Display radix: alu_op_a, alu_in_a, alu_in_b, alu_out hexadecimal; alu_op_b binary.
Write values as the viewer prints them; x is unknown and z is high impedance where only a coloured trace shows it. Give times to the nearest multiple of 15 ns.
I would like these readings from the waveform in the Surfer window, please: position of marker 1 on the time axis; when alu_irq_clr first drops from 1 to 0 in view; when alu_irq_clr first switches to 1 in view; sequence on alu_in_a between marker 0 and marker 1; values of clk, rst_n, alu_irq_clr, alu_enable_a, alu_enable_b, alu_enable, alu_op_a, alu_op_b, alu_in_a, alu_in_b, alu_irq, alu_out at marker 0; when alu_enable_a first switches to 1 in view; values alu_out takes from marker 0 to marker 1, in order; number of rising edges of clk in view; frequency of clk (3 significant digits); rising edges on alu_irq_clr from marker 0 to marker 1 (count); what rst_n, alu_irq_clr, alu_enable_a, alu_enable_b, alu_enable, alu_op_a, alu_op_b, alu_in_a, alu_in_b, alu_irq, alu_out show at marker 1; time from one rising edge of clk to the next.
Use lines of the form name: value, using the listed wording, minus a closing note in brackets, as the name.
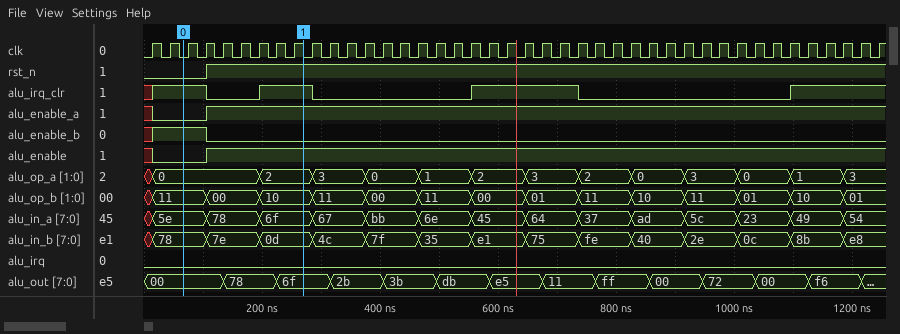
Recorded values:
position of marker 1 on the time axis: 270 ns
when alu_irq_clr first drops from 1 to 0 in view: 105 ns
when alu_irq_clr first switches to 1 in view: 15 ns
sequence on alu_in_a between marker 0 and marker 1: 5e, 78, 6f
values of clk, rst_n, alu_irq_clr, alu_enable_a, alu_enable_b, alu_enable, alu_op_a, alu_op_b, alu_in_a, alu_in_b, alu_irq, alu_out at marker 0: clk=0, rst_n=0, alu_irq_clr=1, alu_enable_a=0, alu_enable_b=1, alu_enable=0, alu_op_a=0, alu_op_b=11, alu_in_a=5e, alu_in_b=78, alu_irq=0, alu_out=00
when alu_enable_a first switches to 1 in view: 105 ns
values alu_out takes from marker 0 to marker 1, in order: 00, 78, 6f
number of rising edges of clk in view: 42
frequency of clk: 33.3 MHz
rising edges on alu_irq_clr from marker 0 to marker 1: 1
what rst_n, alu_irq_clr, alu_enable_a, alu_enable_b, alu_enable, alu_op_a, alu_op_b, alu_in_a, alu_in_b, alu_irq, alu_out show at marker 1: rst_n=1, alu_irq_clr=1, alu_enable_a=1, alu_enable_b=0, alu_enable=1, alu_op_a=2, alu_op_b=10, alu_in_a=6f, alu_in_b=0d, alu_irq=0, alu_out=6f
time from one rising edge of clk to the next: 30 ns
